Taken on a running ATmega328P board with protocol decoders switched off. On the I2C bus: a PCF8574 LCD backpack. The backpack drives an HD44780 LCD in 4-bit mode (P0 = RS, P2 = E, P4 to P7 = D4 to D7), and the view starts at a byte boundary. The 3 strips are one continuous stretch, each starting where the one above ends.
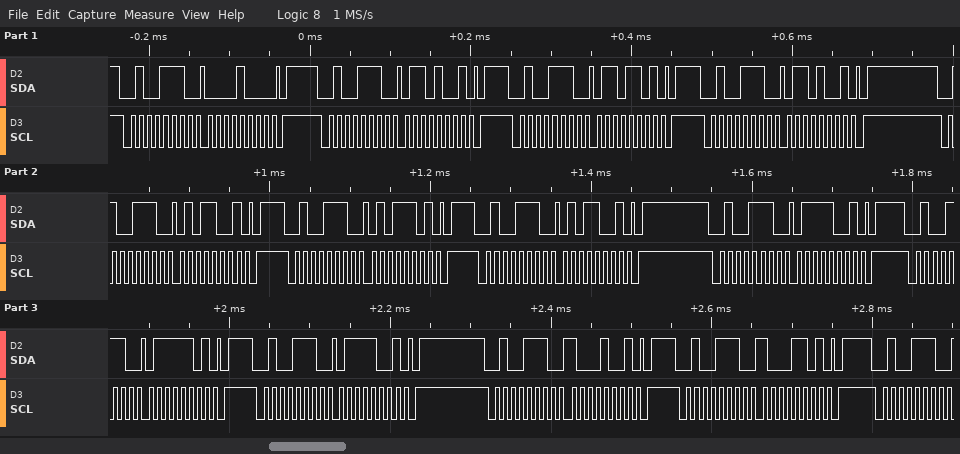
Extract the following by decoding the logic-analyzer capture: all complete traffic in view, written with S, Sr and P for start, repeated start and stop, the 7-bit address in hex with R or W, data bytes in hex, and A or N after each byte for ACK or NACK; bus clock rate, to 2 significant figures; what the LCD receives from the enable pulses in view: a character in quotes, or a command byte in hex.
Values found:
S 27W A 08 A P S 27W A 69 A P S 27W A 6D A P S 27W A 69 A P S 27W A 59 A P S 27W A 5D A P S 27W A 59 A P S 27W A 79 A P S 27W A 7D A P S 27W A 79 A P S 27W A 89 A P S 27W A 8D A P S 27W A
100 kHz
'e'
